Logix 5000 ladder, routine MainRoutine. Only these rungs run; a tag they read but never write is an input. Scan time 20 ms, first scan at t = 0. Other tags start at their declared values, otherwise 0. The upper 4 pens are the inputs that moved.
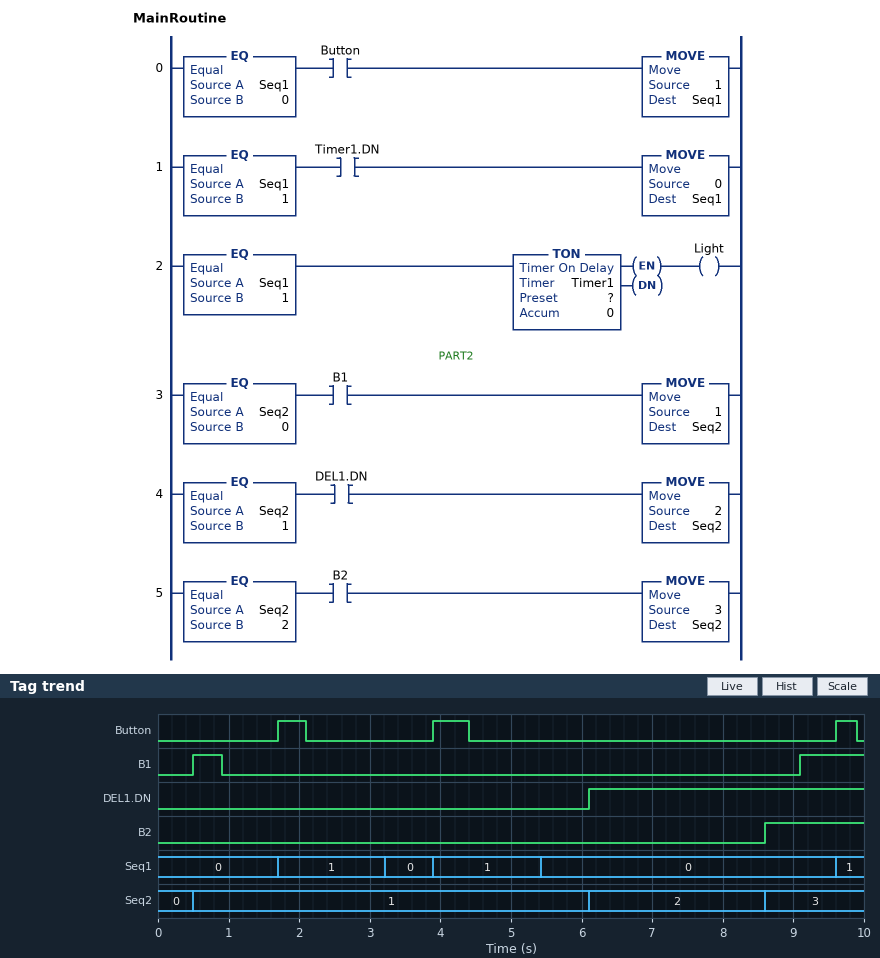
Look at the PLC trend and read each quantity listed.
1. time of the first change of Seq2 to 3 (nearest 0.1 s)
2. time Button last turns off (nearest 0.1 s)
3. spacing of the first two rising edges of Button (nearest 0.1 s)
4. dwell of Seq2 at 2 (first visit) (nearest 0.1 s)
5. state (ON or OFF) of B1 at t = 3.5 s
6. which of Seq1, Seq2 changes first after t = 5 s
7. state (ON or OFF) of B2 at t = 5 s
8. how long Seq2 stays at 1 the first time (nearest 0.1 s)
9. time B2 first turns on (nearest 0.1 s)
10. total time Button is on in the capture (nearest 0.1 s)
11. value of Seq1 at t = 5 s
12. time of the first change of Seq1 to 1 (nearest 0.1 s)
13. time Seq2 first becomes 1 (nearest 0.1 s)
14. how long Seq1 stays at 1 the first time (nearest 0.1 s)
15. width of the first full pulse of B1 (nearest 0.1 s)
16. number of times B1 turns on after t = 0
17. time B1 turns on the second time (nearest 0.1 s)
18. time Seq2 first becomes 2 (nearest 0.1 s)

8.6 s
9.9 s
2.2 s
2.5 s
OFF
Seq1
OFF
5.6 s
8.6 s
1.2 s
1
1.7 s
0.5 s
1.5 s
0.4 s
2
9.1 s
6.1 s
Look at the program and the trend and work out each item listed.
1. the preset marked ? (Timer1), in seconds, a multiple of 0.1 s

1.5 s
